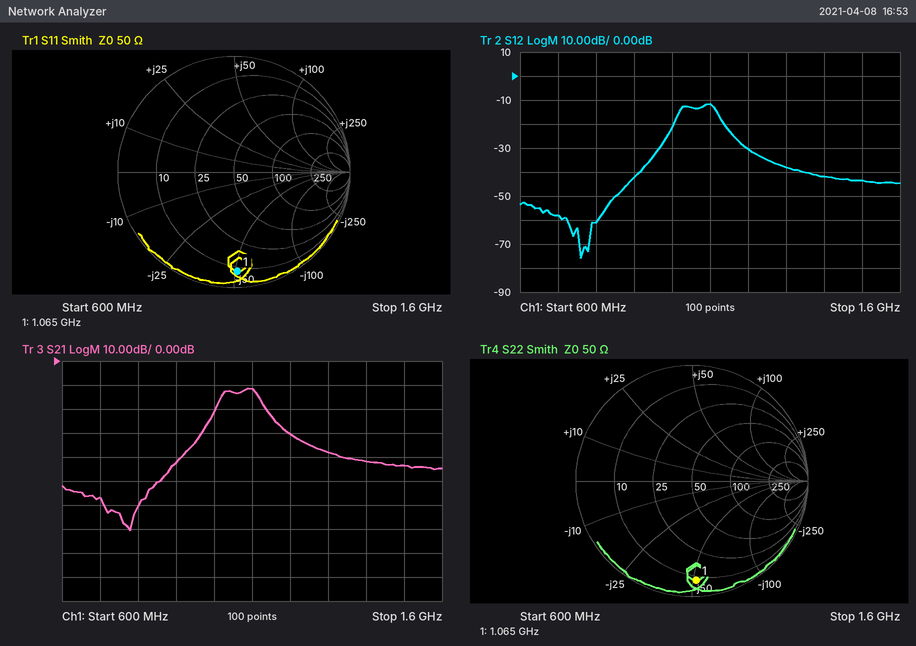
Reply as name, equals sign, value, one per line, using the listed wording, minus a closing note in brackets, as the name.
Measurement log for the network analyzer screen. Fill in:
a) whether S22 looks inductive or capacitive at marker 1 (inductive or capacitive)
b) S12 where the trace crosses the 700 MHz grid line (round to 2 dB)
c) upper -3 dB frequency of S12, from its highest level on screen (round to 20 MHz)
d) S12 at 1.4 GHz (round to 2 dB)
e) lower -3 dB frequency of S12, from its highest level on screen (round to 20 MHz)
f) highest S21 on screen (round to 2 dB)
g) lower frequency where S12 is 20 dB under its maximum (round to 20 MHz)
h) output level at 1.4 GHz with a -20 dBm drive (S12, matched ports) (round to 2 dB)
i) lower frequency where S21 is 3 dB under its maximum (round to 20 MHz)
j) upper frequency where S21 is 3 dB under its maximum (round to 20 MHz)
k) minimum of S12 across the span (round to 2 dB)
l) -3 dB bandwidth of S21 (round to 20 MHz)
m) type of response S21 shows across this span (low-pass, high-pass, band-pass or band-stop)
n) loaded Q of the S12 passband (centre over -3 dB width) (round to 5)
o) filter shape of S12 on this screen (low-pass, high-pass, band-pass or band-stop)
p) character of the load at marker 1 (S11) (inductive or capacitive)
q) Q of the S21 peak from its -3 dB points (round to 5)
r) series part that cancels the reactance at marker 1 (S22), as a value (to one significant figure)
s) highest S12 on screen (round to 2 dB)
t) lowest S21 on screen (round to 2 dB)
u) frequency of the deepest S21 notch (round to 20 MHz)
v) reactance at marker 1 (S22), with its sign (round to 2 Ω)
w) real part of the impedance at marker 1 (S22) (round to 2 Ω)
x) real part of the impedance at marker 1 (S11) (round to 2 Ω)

whether S22 looks inductive or capacitive at marker 1 = capacitive
S12 where the trace crosses the 700 MHz grid line = -58 dB
upper -3 dB frequency of S12, from its highest level on screen = 1.12 GHz
S12 at 1.4 GHz = -42 dB
lower -3 dB frequency of S12, from its highest level on screen = 1.02 GHz
highest S21 on screen = -12 dB
lower frequency where S12 is 20 dB under its maximum = 960 MHz
output level at 1.4 GHz with a -20 dBm drive (S12, matched ports) = -62 dBm
lower frequency where S21 is 3 dB under its maximum = 1.02 GHz
upper frequency where S21 is 3 dB under its maximum = 1.12 GHz
minimum of S12 across the span = -76 dB
-3 dB bandwidth of S21 = 100 MHz
type of response S21 shows across this span = band-pass
loaded Q of the S12 passband (centre over -3 dB width) = 10
filter shape of S12 on this screen = band-pass
character of the load at marker 1 (S11) = capacitive
Q of the S21 peak from its -3 dB points = 10
series part that cancels the reactance at marker 1 (S22), as a value = 8 nH
highest S12 on screen = -12 dB
lowest S21 on screen = -70 dB
frequency of the deepest S21 notch = 780 MHz
reactance at marker 1 (S22), with its sign = -52 Ω
real part of the impedance at marker 1 (S22) = 8 Ω
real part of the impedance at marker 1 (S11) = 8 Ω
